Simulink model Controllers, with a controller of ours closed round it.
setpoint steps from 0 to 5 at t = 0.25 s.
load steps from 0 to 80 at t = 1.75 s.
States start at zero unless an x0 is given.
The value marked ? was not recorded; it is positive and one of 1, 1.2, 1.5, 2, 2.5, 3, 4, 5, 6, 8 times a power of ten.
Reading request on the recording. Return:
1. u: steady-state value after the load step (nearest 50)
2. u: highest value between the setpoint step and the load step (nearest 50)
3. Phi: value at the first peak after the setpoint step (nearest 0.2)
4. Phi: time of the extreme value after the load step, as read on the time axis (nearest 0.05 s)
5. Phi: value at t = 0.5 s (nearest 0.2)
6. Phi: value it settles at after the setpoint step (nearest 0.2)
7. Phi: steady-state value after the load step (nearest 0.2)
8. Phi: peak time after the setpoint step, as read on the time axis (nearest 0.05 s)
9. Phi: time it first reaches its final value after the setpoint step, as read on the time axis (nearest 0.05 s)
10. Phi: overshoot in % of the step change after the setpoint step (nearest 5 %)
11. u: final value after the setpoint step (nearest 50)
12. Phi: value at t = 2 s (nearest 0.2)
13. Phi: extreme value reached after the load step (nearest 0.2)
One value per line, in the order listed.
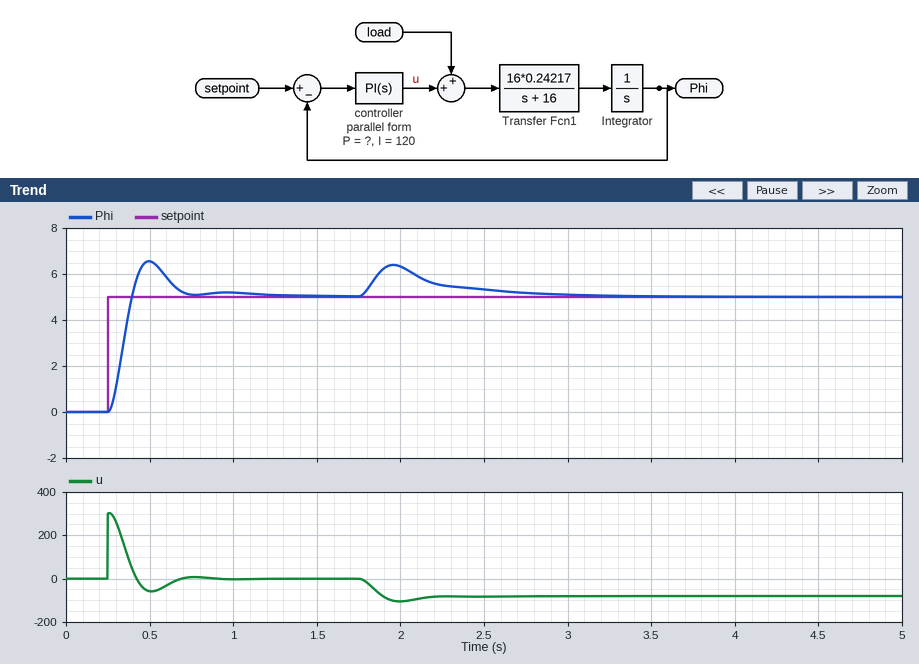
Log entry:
-100
300
6.6
1.95 s
6.6
5.0
5.0
0.50 s
0.40 s
30 %
0
6.4
6.4
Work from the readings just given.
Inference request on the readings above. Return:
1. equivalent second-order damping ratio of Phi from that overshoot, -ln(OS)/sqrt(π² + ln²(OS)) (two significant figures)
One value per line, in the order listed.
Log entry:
0.36
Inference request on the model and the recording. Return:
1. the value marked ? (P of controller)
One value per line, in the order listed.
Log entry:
60
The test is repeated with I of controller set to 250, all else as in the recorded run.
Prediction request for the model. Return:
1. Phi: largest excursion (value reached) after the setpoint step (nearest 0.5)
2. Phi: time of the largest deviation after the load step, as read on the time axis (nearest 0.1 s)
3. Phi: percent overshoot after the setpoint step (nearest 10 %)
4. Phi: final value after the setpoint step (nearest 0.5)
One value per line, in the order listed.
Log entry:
7.5
1.9 s
50 %
5.0
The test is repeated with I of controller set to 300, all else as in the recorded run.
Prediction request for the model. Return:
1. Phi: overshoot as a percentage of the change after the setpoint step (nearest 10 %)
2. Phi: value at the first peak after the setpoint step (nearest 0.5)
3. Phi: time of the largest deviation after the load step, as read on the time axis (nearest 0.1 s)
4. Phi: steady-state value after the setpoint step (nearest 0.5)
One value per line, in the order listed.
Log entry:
50 %
7.5
1.9 s
5.0
